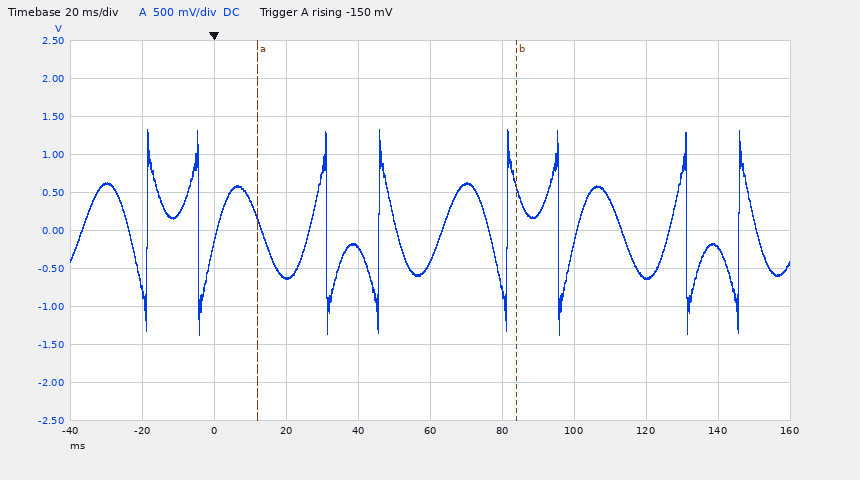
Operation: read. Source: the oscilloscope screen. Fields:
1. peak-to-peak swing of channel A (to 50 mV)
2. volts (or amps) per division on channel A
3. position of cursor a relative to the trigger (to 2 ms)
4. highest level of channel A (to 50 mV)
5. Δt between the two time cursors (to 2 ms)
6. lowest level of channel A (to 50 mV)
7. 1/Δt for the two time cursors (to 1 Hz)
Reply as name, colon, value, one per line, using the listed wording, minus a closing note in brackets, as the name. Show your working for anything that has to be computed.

peak-to-peak swing of channel A: 1.35 V − (-1.35 V) = 2.70 V
volts (or amps) per division on channel A: 500 mV
position of cursor a relative to the trigger: +12 ms
highest level of channel A: 1.35 V
Δt between the two time cursors: 72 ms
lowest level of channel A: -1.35 V
1/Δt for the two time cursors: 1 / 72 ms ≈ 14 Hz
